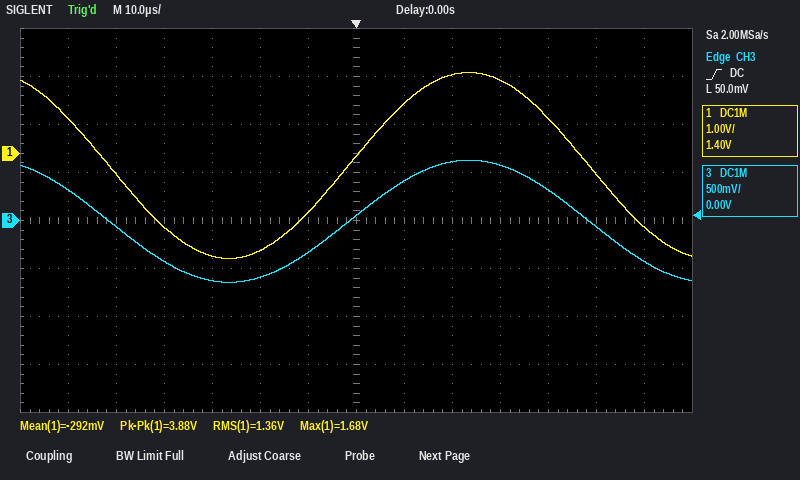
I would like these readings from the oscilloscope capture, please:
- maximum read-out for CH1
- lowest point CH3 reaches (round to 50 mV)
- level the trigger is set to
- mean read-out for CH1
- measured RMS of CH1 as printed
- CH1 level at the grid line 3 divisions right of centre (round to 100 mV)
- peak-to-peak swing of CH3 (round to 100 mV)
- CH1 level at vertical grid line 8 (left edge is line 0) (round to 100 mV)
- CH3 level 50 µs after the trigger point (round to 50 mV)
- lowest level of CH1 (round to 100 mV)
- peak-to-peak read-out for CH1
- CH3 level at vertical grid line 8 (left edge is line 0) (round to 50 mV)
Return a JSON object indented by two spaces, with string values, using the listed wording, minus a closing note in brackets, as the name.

{
  "maximum read-out for CH1": "1.68 V",
  "lowest point CH3 reaches": "-650 mV",
  "level the trigger is set to": "50.0 mV",
  "mean read-out for CH1": "-292 mV",
  "measured RMS of CH1 as printed": "1.36 V",
  "CH1 level at the grid line 3 divisions right of centre": "1.5 V",
  "peak-to-peak swing of CH3": "1.30 V",
  "CH1 level at vertical grid line 8 (left edge is line 0)": "1.0 V",
  "CH3 level 50 µs after the trigger point": "-50 mV",
  "lowest level of CH1": "-2.2 V",
  "peak-to-peak read-out for CH1": "3.88 V",
  "CH3 level at vertical grid line 8 (left edge is line 0)": "400 mV"
}
